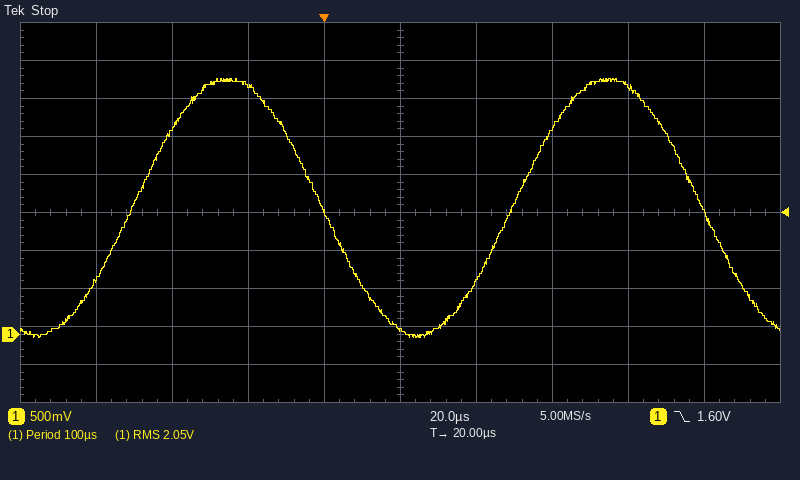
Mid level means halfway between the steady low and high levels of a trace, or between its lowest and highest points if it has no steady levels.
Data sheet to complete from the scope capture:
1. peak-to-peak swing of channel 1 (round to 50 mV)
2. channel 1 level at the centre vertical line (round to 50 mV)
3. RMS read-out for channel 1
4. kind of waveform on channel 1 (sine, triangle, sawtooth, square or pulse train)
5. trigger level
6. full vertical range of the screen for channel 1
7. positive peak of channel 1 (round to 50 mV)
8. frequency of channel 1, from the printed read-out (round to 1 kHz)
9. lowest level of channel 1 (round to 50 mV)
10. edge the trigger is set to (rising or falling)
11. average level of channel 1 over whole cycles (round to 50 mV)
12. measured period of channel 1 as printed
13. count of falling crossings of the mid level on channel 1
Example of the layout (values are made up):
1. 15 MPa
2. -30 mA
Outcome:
1. 3.40 V
2. 100 mV
3. 2.05 V
4. sine
5. 1.60 V
6. 5 V
7. 3.35 V
8. 10 kHz
9. -50 mV
10. falling
11. 1.65 V
12. 100 µs
13. 2
